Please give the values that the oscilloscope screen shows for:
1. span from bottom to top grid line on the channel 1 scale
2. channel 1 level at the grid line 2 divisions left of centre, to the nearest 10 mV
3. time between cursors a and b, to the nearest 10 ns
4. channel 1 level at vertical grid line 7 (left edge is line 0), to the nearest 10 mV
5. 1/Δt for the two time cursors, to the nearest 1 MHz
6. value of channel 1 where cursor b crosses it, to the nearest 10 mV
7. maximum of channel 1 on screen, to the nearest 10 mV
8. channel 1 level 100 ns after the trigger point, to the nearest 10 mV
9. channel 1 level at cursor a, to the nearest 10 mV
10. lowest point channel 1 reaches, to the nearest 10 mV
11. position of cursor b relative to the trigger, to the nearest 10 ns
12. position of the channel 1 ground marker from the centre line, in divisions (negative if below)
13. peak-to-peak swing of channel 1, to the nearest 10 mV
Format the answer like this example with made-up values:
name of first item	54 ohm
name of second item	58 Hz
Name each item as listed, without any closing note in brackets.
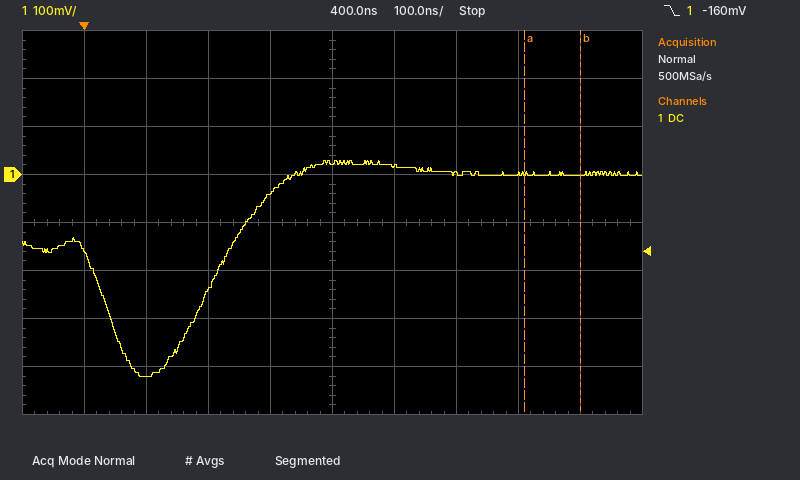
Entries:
span from bottom to top grid line on the channel 1 scale	800 mV
channel 1 level at the grid line 2 divisions left of centre, to the nearest 10 mV	-240 mV
time between cursors a and b, to the nearest 10 ns	90 ns
channel 1 level at vertical grid line 7 (left edge is line 0), to the nearest 10 mV	0 mV
1/Δt for the two time cursors, to the nearest 1 MHz	11 MHz
value of channel 1 where cursor b crosses it, to the nearest 10 mV	0 mV
maximum of channel 1 on screen, to the nearest 10 mV	30 mV
channel 1 level 100 ns after the trigger point, to the nearest 10 mV	-420 mV
channel 1 level at cursor a, to the nearest 10 mV	0 mV
lowest point channel 1 reaches, to the nearest 10 mV	-420 mV
position of cursor b relative to the trigger, to the nearest 10 ns	+800 ns
position of the channel 1 ground marker from the centre line, in divisions	+1.0 div
peak-to-peak swing of channel 1, to the nearest 10 mV	450 mV
